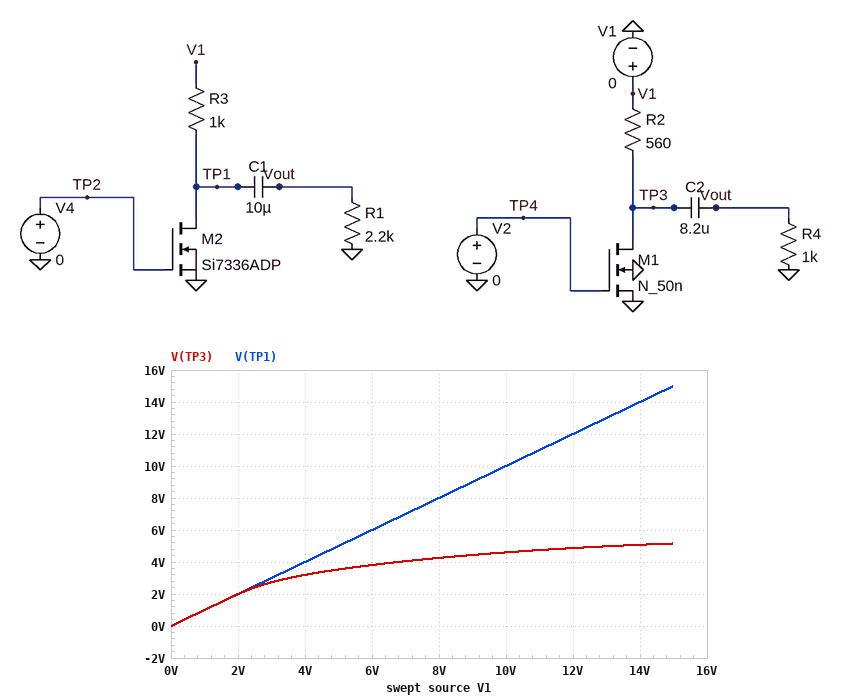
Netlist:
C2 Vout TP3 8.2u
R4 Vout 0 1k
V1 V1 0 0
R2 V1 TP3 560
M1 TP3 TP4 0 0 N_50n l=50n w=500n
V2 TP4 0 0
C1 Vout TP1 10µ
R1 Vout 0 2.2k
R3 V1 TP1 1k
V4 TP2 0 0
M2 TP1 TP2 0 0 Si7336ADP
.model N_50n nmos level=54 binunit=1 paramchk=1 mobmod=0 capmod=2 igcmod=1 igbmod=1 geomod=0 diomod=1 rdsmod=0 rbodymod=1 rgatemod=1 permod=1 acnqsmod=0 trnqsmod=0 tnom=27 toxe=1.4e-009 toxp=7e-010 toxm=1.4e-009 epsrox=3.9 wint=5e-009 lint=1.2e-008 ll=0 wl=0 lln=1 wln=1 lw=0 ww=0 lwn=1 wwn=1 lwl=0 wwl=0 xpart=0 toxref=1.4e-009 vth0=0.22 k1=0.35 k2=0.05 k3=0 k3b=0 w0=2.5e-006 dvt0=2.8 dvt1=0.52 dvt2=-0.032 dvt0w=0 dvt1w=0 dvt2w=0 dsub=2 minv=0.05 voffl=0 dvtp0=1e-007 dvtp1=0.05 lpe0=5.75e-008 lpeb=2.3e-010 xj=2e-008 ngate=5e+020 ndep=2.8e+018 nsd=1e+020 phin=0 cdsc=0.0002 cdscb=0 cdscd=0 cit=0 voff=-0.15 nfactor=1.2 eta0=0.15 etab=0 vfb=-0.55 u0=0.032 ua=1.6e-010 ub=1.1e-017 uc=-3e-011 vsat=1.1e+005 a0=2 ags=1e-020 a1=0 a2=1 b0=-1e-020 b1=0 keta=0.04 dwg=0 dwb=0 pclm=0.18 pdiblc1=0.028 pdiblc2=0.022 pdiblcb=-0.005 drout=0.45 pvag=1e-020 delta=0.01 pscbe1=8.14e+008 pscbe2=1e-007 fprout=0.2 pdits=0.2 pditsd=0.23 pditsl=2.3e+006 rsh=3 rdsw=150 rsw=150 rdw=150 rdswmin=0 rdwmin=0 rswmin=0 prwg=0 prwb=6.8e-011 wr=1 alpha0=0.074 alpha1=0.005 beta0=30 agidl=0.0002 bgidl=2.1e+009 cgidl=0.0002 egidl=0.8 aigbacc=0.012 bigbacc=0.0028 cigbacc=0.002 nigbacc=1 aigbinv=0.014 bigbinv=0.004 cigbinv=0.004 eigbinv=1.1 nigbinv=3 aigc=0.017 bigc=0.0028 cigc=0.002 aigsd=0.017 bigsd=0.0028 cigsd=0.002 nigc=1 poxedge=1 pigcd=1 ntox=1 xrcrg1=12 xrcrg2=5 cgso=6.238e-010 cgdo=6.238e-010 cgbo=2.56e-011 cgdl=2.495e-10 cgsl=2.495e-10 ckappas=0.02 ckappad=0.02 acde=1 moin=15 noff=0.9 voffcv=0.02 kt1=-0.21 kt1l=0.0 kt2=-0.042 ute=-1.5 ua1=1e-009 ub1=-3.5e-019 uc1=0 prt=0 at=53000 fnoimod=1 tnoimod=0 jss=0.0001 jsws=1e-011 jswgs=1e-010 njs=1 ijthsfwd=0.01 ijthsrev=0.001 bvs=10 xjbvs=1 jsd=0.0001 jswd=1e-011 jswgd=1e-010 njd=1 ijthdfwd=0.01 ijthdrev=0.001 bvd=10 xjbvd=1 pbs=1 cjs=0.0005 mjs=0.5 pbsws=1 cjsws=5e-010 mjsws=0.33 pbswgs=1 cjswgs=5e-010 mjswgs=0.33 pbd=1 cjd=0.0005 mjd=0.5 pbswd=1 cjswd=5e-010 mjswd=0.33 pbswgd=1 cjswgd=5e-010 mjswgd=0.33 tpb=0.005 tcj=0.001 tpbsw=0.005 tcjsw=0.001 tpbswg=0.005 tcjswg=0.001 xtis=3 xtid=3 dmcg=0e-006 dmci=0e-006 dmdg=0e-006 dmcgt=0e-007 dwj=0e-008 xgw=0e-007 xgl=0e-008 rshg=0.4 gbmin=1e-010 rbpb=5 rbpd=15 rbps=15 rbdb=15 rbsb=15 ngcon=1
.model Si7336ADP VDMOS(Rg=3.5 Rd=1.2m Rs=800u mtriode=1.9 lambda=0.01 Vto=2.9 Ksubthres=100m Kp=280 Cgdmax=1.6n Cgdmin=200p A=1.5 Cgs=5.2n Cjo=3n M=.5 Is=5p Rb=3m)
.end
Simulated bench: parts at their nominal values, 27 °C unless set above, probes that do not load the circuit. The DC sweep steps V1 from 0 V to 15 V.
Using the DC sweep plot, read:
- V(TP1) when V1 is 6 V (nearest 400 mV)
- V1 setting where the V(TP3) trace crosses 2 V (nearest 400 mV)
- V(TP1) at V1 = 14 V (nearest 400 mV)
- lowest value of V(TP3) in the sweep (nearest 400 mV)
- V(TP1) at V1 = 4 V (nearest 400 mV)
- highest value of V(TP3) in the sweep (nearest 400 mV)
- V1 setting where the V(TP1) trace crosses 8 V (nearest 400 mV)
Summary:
6.0 V
2.0 V
14.0 V
0 V
4.0 V
5.2 V
8.0 V
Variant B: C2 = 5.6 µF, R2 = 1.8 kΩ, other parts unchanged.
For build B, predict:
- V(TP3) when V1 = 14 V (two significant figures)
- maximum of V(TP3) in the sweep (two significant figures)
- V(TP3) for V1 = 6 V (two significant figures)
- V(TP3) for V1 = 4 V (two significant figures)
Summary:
4.1 V
4.2 V
3.2 V
2.8 V
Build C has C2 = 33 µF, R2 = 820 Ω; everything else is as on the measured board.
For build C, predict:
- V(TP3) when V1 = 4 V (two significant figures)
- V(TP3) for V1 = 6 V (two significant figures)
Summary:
3.1 V
3.6 V
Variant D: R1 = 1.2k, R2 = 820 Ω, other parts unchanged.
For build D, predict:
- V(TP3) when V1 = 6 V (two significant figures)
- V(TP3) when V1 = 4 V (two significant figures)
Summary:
3.6 V
3.1 V
